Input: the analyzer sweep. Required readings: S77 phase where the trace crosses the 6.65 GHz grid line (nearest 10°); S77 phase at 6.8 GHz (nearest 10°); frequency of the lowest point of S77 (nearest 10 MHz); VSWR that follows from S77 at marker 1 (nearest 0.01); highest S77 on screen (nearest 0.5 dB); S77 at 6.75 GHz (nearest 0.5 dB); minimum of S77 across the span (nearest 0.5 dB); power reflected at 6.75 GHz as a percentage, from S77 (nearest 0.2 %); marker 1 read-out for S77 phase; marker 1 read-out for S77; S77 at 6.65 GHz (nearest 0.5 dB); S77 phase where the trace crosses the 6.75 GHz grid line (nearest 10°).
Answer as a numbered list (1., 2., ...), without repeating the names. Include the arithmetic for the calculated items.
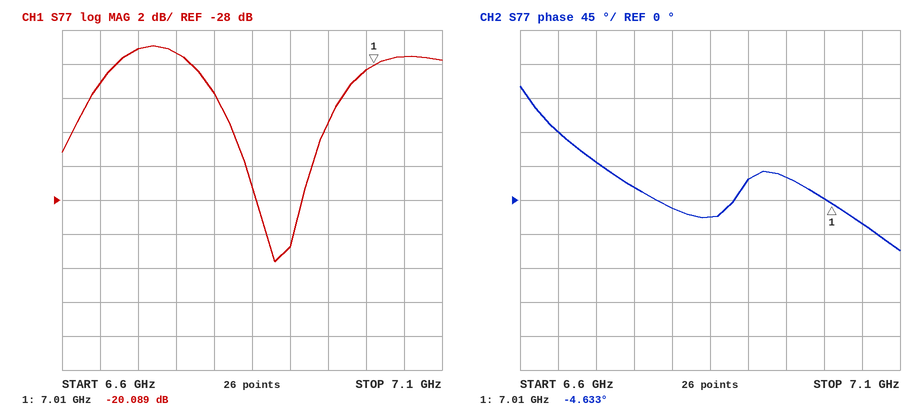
1. 90°
2. -10°
3. 6.88 GHz
4. (1 + 0.0990)/(1 − 0.0990) ≈ 1.22
5. -19.0 dB
6. -19.5 dB
7. -31.5 dB
8. 10^(-19.5/10) ≈ 1.12 %, so 1.2 % to the nearest 0.2 %
9. -4.633°
10. -20.089 dB
11. -21.0 dB
12. 20°
